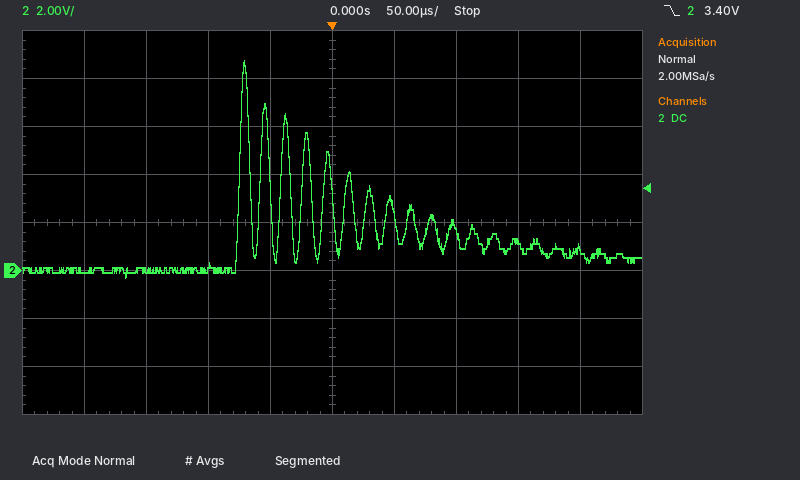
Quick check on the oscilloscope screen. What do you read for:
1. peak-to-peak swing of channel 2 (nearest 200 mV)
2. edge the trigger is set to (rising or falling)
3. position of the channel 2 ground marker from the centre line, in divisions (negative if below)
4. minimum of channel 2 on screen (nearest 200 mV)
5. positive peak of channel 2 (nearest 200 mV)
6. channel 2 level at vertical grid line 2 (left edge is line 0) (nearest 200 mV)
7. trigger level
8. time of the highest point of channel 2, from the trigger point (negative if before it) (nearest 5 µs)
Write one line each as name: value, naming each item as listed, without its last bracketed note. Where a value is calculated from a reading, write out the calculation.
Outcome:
peak-to-peak swing of channel 2: 8.8 V − (-200 mV) = 9.0 V
edge the trigger is set to: falling
position of the channel 2 ground marker from the centre line, in divisions: -1.0 div
minimum of channel 2 on screen: -200 mV
positive peak of channel 2: 8.8 V
channel 2 level at vertical grid line 2 (left edge is line 0): 0.0 V
trigger level: 3.40 V
time of the highest point of channel 2, from the trigger point (negative if before it): -70 µs
